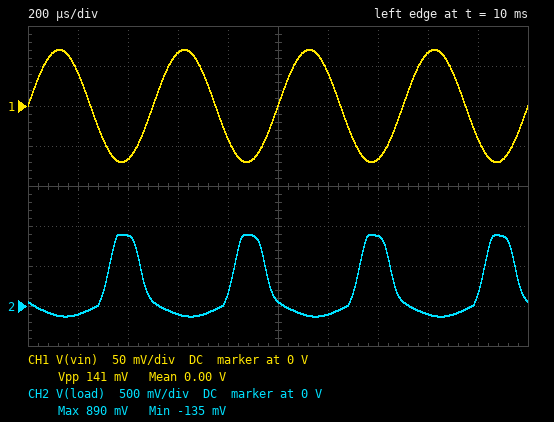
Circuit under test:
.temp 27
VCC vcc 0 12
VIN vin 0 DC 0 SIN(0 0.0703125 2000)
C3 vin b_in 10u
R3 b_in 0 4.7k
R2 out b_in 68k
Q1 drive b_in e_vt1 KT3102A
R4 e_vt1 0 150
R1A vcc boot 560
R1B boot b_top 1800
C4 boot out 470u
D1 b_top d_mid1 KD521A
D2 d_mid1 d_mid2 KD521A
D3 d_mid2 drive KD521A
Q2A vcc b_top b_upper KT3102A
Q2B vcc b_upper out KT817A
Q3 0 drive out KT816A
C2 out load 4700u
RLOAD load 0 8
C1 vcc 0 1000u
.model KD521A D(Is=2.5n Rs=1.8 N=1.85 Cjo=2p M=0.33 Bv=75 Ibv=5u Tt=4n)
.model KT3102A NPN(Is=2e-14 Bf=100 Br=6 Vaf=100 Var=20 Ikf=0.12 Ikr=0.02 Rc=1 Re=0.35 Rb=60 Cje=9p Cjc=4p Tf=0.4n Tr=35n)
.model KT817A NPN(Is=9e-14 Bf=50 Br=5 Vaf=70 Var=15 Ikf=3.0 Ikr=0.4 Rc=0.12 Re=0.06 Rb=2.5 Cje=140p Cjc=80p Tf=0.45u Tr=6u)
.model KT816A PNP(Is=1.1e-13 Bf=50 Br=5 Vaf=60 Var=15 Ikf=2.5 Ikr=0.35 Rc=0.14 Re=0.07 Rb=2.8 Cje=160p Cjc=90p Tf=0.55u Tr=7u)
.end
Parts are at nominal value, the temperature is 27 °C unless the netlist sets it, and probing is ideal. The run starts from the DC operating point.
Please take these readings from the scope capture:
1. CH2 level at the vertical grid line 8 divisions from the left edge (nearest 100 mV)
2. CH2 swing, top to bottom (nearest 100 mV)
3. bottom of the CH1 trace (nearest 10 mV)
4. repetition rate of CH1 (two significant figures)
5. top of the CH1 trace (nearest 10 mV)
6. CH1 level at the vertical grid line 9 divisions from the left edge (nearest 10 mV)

-100 mV
1.0 V
-70 mV
2.0 kHz
70 mV
-40 mV
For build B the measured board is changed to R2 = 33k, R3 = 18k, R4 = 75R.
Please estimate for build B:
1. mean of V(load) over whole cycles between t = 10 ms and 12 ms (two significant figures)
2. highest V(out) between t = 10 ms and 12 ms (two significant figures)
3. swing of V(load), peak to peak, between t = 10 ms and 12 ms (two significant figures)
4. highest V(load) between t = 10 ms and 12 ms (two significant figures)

67 mV
4.8 V
1.2 V
810 mV
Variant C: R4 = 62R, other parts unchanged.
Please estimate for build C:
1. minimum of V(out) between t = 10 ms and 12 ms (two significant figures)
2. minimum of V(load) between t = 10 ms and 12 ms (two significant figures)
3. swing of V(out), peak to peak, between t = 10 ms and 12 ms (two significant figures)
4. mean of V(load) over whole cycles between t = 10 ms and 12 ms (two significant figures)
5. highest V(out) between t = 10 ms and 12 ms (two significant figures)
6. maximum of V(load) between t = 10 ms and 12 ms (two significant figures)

9.8 V
-290 mV
1.4 V
300 mV
11 V
1.1 V
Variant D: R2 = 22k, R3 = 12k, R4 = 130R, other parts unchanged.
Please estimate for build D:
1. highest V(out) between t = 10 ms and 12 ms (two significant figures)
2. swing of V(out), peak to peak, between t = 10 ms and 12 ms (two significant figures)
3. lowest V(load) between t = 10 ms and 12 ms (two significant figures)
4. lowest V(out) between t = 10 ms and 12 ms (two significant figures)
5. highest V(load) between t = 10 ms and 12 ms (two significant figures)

4.4 V
590 mV
-250 mV
3.8 V
340 mV
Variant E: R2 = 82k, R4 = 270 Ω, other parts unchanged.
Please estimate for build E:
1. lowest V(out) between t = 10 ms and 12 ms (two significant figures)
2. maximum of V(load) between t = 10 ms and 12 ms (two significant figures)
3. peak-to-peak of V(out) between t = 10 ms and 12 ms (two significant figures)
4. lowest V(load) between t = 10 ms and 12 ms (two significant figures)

11 V
7.0 mV
44 mV
-37 mV
